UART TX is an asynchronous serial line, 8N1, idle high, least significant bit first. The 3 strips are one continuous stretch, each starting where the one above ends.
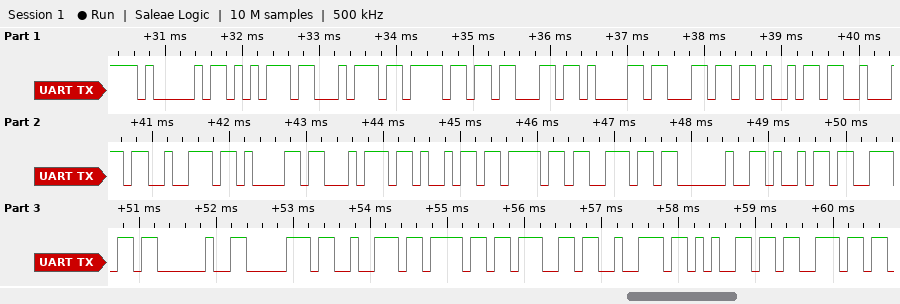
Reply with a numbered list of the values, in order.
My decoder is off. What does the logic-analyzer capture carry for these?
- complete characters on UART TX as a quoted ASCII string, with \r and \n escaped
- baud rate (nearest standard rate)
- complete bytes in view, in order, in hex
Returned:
1. "Autocalibration in progres"
2. 9600 baud
3. 41 75 74 6F 63 61 6C 69 62 72 61 74 69 6F 6E 20 69 6E 20 70 72 6F 67 72 65 73
